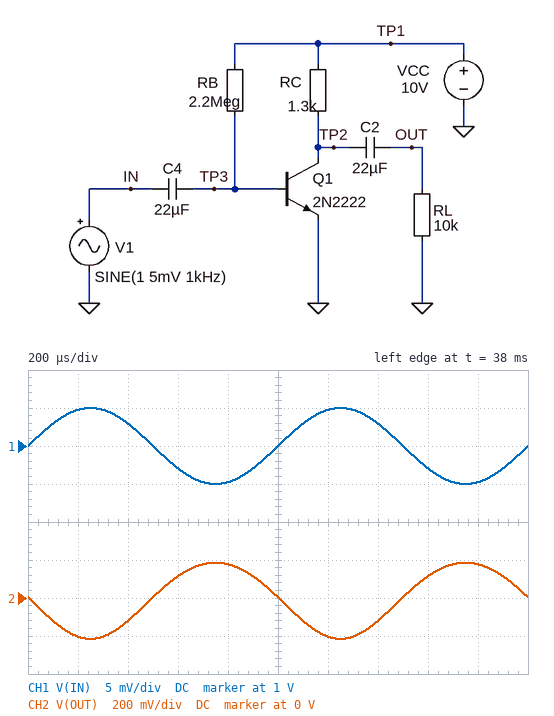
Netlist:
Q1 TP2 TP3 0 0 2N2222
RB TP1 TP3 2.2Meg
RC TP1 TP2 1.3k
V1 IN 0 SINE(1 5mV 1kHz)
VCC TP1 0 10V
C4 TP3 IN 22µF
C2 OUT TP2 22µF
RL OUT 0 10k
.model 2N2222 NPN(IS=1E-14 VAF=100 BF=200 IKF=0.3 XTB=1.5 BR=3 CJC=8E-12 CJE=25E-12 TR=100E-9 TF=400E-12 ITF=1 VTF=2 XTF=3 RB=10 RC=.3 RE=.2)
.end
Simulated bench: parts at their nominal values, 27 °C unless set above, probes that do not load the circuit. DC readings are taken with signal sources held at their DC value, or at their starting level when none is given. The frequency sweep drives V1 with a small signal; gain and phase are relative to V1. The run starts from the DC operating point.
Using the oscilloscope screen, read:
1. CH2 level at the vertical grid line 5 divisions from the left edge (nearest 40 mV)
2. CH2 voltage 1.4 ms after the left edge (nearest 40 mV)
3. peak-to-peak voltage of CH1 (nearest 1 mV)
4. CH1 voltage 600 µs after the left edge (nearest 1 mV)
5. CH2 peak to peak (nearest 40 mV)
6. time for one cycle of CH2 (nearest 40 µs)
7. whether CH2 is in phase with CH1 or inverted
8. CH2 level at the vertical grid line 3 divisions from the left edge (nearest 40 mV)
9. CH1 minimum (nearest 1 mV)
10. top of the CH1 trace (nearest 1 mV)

0 V
-120 mV
10 mV
997 mV
400 mV
1.00 ms
inverted
120 mV
995 mV
1.005 V
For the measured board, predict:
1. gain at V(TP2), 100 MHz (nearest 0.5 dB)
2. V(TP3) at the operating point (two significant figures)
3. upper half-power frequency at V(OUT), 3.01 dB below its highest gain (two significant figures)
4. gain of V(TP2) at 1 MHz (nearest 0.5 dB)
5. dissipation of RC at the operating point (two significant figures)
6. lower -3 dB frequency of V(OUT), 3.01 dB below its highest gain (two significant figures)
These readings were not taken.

20.5 dB
650 mV
28 MHz
32.0 dB
1.1 mW
1.4 Hz
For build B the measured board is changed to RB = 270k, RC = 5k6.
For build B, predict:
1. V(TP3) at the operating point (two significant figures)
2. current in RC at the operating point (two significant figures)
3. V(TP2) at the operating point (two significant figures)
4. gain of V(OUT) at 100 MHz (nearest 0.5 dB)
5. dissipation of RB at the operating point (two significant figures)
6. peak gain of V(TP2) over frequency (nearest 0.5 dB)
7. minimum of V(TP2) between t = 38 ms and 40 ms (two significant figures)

670 mV
1.8 mA
84 mV
-4.5 dB
320 µW
23.0 dB
58 mV
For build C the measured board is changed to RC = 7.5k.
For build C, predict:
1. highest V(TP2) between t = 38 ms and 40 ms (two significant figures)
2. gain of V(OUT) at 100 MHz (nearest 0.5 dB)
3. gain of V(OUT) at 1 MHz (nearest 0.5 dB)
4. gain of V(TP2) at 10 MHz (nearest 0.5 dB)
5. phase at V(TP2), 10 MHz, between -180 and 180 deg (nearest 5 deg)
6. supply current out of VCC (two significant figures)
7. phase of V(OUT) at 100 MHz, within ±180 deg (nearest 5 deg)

4.1 V
18.0 dB
42.5 dB
37.0 dB
120 deg
880 µA
75 deg
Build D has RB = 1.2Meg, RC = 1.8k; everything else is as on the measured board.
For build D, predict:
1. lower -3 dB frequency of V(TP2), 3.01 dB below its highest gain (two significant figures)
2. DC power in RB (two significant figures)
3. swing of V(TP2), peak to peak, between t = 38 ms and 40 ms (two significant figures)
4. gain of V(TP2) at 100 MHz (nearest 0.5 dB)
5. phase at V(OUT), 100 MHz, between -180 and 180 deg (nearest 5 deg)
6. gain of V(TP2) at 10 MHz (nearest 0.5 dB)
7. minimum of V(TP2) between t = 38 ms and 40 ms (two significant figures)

2.1 Hz
73 µW
930 mV
23.5 dB
85 deg
38.0 dB
6.5 V
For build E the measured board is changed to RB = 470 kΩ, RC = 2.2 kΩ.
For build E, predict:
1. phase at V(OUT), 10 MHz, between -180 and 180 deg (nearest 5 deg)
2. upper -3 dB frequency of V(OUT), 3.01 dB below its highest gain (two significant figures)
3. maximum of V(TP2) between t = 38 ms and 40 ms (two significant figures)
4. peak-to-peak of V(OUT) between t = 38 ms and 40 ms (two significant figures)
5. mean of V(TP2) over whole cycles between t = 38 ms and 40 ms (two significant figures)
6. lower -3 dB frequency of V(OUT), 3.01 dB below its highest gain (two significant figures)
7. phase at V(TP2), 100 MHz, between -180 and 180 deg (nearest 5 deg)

120 deg
5.8 MHz
2.6 V
2.4 V
1.4 V
5.4 Hz
80 deg
